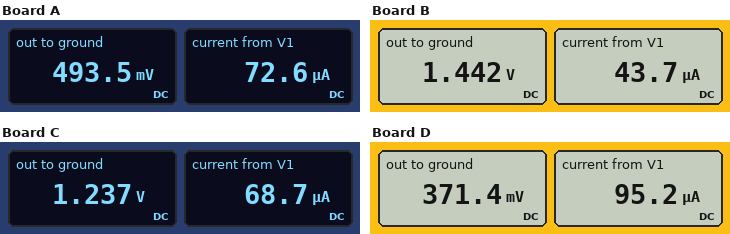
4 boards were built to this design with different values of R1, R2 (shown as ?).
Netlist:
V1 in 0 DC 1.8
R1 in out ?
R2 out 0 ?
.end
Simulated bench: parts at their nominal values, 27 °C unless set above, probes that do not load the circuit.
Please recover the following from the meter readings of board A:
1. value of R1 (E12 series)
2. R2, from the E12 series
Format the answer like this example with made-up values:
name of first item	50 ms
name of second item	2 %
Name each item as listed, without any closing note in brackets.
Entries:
value of R1	18 kΩ
R2, from the E12 series	6.8 kΩ
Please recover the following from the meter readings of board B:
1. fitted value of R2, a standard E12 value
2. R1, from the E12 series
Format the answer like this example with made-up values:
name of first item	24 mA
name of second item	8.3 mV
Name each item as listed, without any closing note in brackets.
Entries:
fitted value of R2, a standard E12 value	33 kΩ
R1, from the E12 series	8.2 kΩ
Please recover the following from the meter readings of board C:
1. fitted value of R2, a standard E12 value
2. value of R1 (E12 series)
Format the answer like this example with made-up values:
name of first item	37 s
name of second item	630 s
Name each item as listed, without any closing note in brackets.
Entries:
fitted value of R2, a standard E12 value	18 kΩ
value of R1	8.2 kΩ
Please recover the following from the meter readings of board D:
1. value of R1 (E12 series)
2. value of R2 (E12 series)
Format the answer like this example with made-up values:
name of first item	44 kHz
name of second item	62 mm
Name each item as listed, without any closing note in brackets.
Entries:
value of R1	15 kΩ
value of R2	3.9 kΩ
